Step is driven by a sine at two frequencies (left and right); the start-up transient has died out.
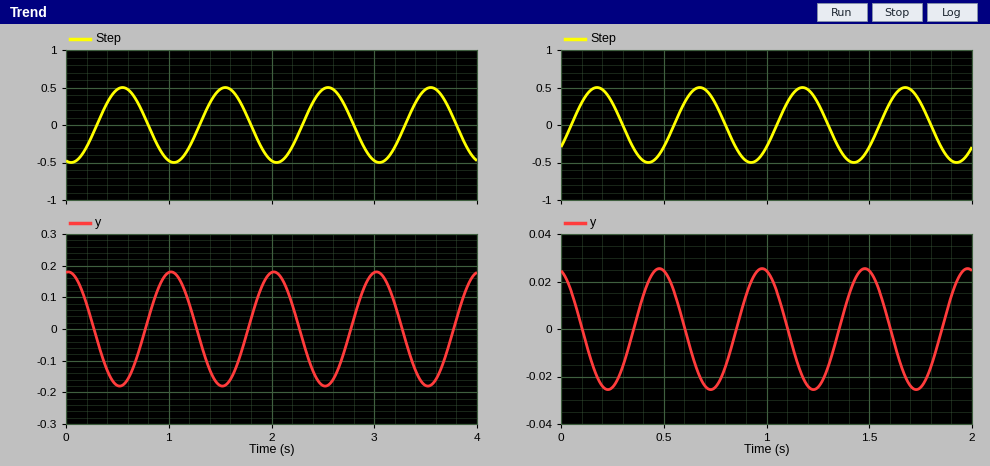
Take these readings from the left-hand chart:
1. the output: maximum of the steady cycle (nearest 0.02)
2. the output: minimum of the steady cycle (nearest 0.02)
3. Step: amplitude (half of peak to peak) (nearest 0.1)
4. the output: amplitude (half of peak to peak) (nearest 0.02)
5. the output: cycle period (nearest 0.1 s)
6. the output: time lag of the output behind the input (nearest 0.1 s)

0.18
-0.18
0.5
0.18
1.0 s
0.5 s
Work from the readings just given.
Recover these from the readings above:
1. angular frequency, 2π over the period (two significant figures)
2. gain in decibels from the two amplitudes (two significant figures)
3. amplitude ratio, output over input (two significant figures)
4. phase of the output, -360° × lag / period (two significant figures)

6.3 rad/s
-8.9 dB
0.36
-180°
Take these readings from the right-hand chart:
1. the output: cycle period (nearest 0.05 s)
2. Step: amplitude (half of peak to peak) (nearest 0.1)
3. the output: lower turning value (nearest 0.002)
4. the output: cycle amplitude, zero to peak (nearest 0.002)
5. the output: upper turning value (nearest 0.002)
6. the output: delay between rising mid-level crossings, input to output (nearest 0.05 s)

0.50 s
0.5
-0.026
0.026
0.026
0.30 s
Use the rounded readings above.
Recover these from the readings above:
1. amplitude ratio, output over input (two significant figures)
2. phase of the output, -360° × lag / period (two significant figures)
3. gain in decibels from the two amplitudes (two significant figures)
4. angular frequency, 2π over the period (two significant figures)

0.052
-220°
-26 dB
13 rad/s
